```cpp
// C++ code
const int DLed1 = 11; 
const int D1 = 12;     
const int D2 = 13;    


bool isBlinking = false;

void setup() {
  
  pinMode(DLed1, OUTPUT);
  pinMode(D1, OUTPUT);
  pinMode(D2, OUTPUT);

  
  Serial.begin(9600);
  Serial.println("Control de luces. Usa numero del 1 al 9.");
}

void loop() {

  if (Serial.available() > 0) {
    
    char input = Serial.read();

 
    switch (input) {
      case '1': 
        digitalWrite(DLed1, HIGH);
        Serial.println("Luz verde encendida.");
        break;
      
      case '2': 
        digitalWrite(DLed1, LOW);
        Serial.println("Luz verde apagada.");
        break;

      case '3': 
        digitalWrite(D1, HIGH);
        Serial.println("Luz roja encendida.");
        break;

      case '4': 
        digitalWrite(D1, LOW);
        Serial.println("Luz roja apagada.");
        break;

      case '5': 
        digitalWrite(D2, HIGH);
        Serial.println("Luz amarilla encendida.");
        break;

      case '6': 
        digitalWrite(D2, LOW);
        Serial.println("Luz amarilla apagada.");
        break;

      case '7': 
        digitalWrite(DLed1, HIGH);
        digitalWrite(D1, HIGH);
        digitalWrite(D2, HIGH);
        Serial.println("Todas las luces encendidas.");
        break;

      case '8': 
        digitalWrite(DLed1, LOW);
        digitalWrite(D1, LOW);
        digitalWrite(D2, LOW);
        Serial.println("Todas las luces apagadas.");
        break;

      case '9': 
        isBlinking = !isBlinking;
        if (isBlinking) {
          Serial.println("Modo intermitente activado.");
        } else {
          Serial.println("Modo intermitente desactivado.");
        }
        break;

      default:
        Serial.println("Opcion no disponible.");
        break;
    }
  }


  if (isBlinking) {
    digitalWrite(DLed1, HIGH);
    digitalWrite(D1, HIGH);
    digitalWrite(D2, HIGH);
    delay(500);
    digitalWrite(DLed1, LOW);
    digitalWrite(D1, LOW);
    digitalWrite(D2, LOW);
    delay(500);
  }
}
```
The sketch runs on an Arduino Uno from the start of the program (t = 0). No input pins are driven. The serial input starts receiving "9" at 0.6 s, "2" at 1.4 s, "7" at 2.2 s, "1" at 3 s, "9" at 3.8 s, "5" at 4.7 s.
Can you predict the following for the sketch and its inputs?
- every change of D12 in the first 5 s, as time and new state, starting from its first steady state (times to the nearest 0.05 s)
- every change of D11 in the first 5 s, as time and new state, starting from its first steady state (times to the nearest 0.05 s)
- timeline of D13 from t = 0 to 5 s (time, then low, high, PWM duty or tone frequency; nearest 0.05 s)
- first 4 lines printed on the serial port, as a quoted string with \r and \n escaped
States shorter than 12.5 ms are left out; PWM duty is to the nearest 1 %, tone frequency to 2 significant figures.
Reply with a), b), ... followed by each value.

a) 0 s low; 0.6 s high; 1.1 s low; 1.6 s high; 2.1 s low; 2.6 s high; 3.1 s low; 3.6 s high; 4.1 s low
b) 0 s low; 0.6 s high; 1.1 s low; 1.6 s high; 2.1 s low; 2.6 s high; 3.1 s low; 3.6 s high; 4.1 s low
c) 0 s low; 0.6 s high; 1.1 s low; 1.6 s high; 2.1 s low; 2.6 s high; 3.1 s low; 3.6 s high; 4.1 s low; 4.7 s high
d) "Control de luces. Usa numero del 1 al 9.\r\nModo intermitente activado.\r\nLuz verde apagada.\r\nTodas las luces encendidas.\r\n"
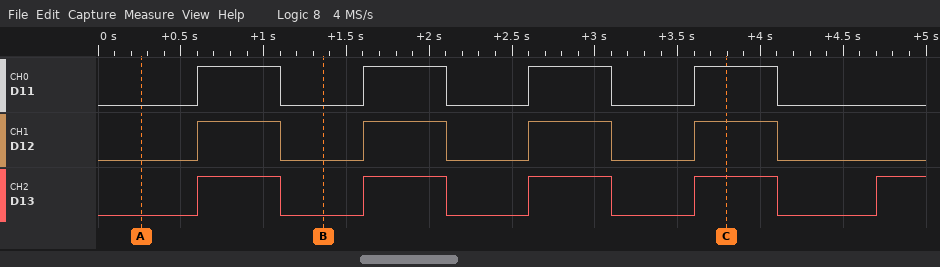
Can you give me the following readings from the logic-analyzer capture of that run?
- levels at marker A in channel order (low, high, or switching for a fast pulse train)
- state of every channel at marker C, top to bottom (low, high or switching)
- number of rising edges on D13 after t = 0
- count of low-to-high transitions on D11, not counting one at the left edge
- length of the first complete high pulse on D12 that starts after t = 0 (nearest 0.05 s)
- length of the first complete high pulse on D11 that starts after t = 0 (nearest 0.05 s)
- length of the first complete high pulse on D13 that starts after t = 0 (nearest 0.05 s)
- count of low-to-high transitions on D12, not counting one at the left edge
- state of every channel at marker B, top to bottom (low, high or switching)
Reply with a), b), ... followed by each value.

a) D11 low, D12 low, D13 low
b) D11 high, D12 high, D13 high
c) 5
d) 4
e) 0.50 s
f) 0.50 s
g) 0.50 s
h) 4
i) D11 low, D12 low, D13 low
